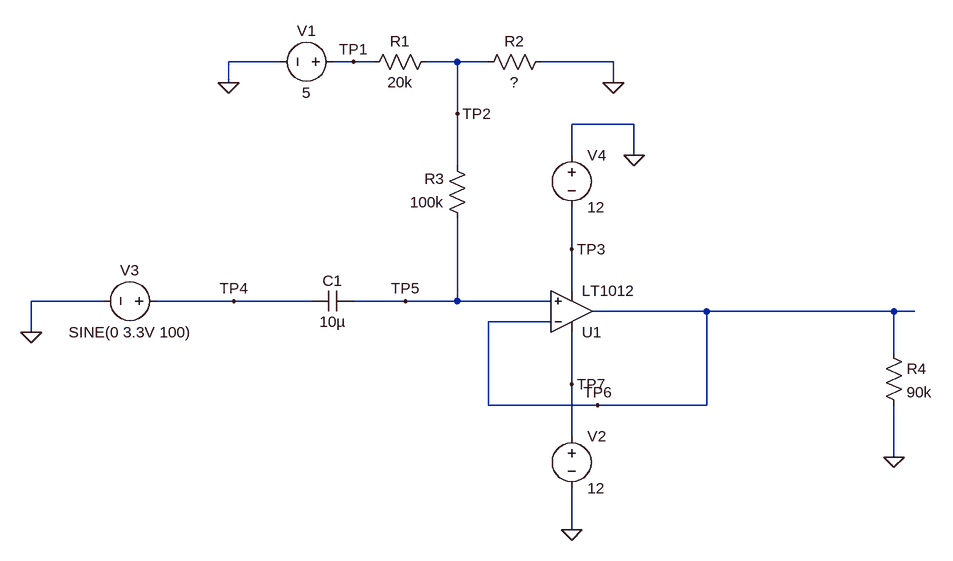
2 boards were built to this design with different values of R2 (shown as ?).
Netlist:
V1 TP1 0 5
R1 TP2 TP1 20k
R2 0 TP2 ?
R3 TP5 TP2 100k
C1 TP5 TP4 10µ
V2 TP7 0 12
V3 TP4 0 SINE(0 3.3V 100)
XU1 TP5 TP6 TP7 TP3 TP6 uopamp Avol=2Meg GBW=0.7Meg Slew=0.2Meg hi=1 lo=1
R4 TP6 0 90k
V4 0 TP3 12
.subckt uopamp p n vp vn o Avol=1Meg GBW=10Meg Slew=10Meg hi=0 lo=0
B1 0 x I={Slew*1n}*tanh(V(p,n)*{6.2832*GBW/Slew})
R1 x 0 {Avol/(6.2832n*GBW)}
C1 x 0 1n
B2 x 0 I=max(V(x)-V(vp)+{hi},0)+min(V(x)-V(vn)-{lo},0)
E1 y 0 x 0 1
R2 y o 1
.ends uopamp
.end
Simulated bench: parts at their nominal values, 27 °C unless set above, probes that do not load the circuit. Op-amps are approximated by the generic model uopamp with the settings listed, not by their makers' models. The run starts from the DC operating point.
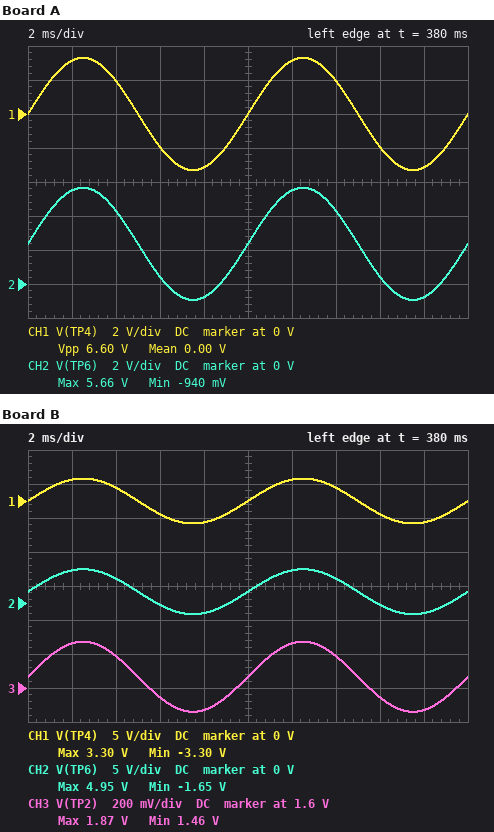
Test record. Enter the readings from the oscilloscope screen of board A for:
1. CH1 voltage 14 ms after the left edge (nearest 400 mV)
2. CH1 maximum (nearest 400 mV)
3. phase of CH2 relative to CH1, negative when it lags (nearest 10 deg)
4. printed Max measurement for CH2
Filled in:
2.0 V
3.2 V
0 deg
5.66 V
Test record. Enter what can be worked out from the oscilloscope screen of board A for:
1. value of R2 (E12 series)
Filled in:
18 kΩ
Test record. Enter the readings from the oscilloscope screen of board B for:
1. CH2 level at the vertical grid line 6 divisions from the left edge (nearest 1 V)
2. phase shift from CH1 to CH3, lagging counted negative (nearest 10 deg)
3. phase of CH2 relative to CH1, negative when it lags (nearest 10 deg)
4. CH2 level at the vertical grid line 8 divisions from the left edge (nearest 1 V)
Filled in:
5 V
0 deg
0 deg
0 V
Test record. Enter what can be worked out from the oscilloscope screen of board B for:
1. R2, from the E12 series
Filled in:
10 kΩ
